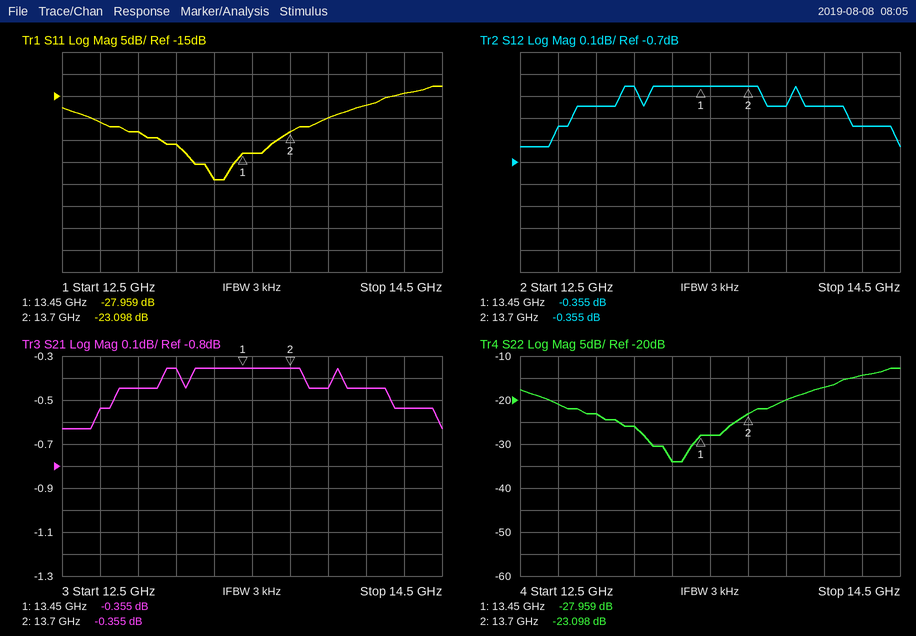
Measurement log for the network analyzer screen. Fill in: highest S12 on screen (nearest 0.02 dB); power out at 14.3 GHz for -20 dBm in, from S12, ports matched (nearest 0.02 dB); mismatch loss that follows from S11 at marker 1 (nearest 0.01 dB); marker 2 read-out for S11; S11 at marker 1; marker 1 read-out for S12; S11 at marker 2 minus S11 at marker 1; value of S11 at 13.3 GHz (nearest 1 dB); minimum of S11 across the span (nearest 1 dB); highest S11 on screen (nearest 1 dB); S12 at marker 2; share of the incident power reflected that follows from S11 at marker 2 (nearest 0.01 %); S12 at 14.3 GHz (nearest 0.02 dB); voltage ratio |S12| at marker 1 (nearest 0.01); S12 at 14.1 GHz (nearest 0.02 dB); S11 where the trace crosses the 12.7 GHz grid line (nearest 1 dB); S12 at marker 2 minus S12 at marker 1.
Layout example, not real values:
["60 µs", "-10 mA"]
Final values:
["-0.36 dB", "-20.54 dBm", "0.01 dB", "-23.098 dB", "-27.959 dB", "-0.355 dB", "4.861 dB", "-34 dB", "-34 dB", "-13 dB", "-0.355 dB", "0.49 %", "-0.54 dB", "0.96", "-0.44 dB", "-21 dB", "0.000 dB"]
